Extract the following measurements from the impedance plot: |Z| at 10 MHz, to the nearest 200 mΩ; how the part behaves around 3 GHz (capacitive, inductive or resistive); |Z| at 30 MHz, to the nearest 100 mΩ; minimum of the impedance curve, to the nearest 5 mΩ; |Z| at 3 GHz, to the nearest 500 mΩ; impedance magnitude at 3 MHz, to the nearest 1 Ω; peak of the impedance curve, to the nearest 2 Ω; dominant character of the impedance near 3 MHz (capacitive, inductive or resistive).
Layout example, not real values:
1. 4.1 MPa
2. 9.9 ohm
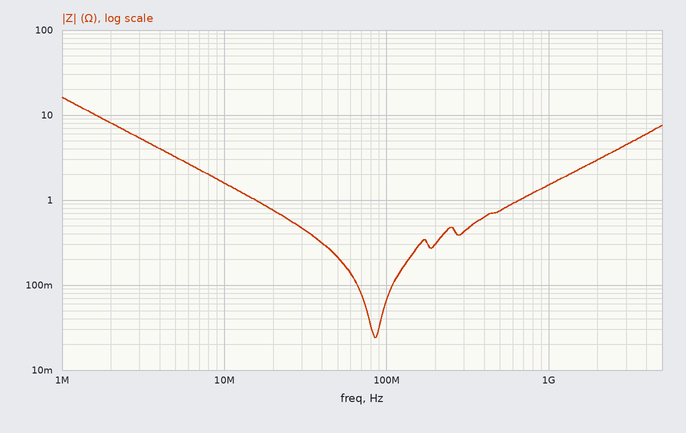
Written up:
1. 1.6 Ω
2. inductive
3. 500 mΩ
4. 25 mΩ
5. 4.5 Ω
6. 5 Ω
7. 16 Ω
8. capacitive
